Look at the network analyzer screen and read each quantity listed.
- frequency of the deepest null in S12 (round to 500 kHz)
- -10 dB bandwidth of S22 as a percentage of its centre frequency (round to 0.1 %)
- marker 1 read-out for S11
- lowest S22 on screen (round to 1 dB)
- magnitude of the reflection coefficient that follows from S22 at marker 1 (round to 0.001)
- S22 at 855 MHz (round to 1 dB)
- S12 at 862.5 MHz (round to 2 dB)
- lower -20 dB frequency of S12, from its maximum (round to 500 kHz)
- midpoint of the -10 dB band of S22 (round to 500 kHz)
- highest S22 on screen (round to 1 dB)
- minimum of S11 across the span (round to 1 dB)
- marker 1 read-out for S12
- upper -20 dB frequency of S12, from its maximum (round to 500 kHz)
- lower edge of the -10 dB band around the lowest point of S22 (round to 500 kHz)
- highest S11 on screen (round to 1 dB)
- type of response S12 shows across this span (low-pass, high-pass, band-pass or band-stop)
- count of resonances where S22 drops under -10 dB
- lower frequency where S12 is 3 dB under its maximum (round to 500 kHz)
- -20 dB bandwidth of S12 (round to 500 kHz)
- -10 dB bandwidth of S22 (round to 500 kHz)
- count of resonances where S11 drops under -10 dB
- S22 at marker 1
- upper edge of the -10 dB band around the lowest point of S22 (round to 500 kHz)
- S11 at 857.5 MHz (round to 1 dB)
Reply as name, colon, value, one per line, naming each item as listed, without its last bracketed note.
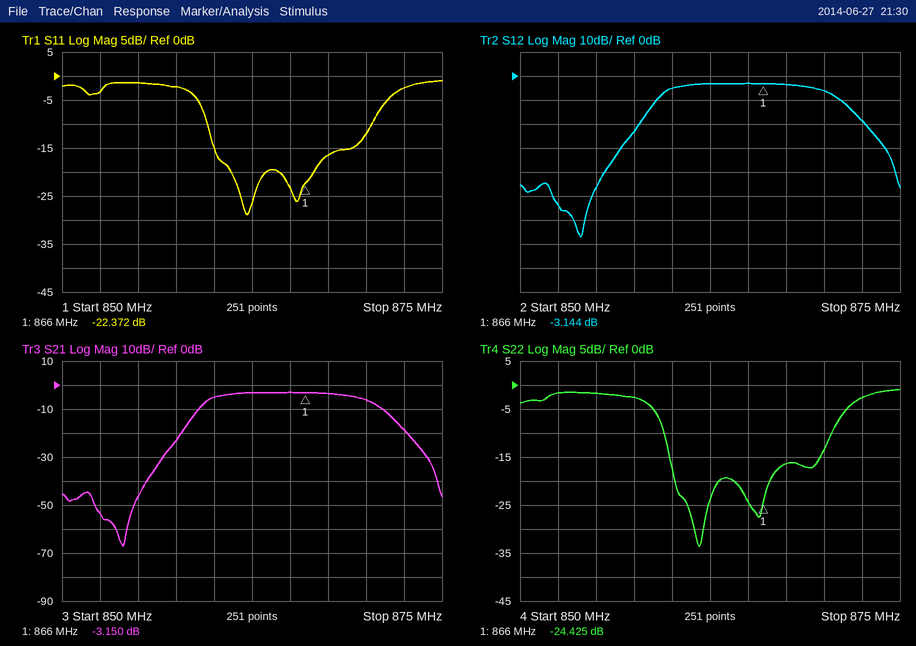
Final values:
frequency of the deepest null in S12: 854.0 MHz
-10 dB bandwidth of S22 as a percentage of its centre frequency: 1.3 %
marker 1 read-out for S11: -22.372 dB
lowest S22 on screen: -34 dB
magnitude of the reflection coefficient that follows from S22 at marker 1: 0.060
S22 at 855 MHz: -2 dB
S12 at 862.5 MHz: -4 dB
lower -20 dB frequency of S12, from its maximum: 857.5 MHz
midpoint of the -10 dB band of S22: 865.0 MHz
highest S22 on screen: -1 dB
minimum of S11 across the span: -29 dB
marker 1 read-out for S12: -3.144 dB
upper -20 dB frequency of S12, from its maximum: 873.0 MHz
lower edge of the -10 dB band around the lowest point of S22: 859.5 MHz
highest S11 on screen: -1 dB
type of response S12 shows across this span: band-pass
count of resonances where S22 drops under -10 dB: 2
lower frequency where S12 is 3 dB under its maximum: 859.5 MHz
-20 dB bandwidth of S12: 15.5 MHz
-10 dB bandwidth of S22: 11.0 MHz
count of resonances where S11 drops under -10 dB: 2
S22 at marker 1: -24.425 dB
upper edge of the -10 dB band around the lowest point of S22: 870.5 MHz
S11 at 857.5 MHz: -2 dB
